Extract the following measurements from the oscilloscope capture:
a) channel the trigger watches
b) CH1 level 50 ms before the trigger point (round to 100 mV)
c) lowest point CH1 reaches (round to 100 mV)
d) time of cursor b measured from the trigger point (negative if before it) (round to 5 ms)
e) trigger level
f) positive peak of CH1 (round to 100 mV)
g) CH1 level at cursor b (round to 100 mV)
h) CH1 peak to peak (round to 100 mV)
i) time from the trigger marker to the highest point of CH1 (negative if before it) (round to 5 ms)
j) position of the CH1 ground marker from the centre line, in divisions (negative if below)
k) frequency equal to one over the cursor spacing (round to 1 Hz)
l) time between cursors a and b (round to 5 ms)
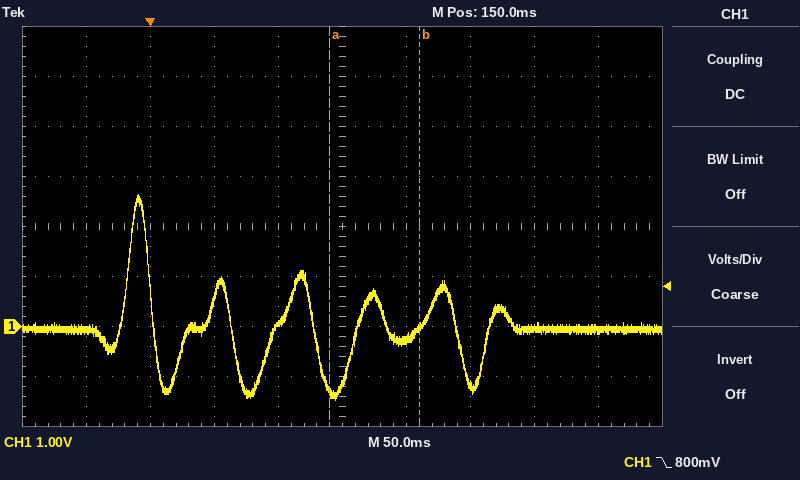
CH1
-100 mV
-1.5 V
+210 ms
800 mV
2.6 V
0.0 V
4.1 V
-10 ms
-2.0 div
14 Hz
70 ms
